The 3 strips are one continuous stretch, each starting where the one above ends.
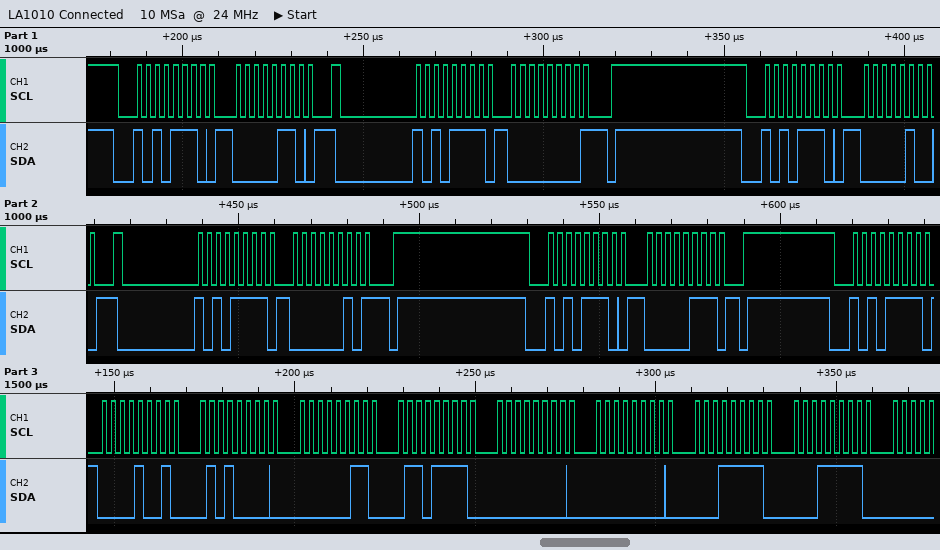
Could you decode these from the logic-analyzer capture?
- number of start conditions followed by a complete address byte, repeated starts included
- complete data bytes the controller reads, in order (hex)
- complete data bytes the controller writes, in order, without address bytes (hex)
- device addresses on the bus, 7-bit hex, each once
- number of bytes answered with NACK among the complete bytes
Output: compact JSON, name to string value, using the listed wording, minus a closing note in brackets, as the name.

{"number of start conditions followed by a complete address byte, repeated starts included": "6", "complete data bytes the controller reads, in order": "00 02 09 50 03 6F 00 00 1F 1F", "complete data bytes the controller writes, in order, without address bytes": "06 04 07", "device addresses on the bus, 7-bit hex, each once": "0x57", "number of bytes answered with NACK among the complete bytes": "2"}
